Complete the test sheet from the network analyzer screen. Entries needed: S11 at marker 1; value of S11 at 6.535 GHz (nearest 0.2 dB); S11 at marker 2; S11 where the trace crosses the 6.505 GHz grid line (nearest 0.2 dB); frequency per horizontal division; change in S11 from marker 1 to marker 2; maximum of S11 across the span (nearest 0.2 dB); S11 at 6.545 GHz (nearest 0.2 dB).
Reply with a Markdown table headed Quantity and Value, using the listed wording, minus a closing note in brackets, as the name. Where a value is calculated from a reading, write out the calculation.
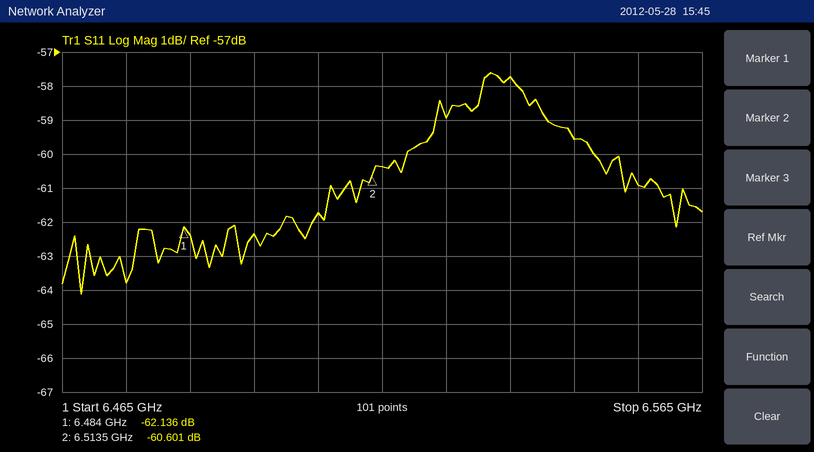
| Quantity | Value |
|---|---|
| S11 at marker 1 | -62.136 dB |
| value of S11 at 6.535 GHz | -57.8 dB |
| S11 at marker 2 | -60.601 dB |
| S11 where the trace crosses the 6.505 GHz grid line | -61.8 dB |
| frequency per horizontal division | 10 MHz |
| change in S11 from marker 1 to marker 2 | -60.601 − (-62.136) = 1.535 dB |
| maximum of S11 across the span | -57.6 dB |
| S11 at 6.545 GHz | -59.6 dB |
